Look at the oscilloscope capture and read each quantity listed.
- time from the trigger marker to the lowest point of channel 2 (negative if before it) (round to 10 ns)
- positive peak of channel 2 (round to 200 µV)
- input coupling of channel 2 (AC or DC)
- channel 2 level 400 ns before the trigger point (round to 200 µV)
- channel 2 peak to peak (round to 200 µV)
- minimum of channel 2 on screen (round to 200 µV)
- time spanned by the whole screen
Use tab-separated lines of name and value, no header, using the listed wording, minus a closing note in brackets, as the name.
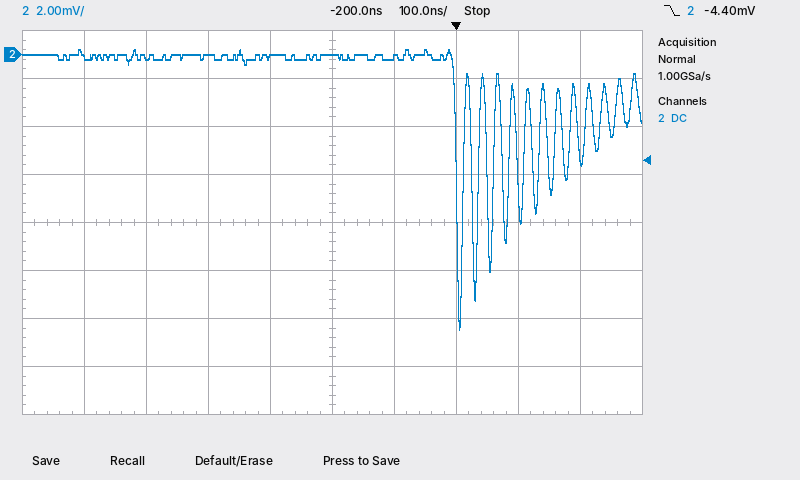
time from the trigger marker to the lowest point of channel 2 (negative if before it)	+10 ns
positive peak of channel 2	200 µV
input coupling of channel 2	DC
channel 2 level 400 ns before the trigger point	0.0 mV
channel 2 peak to peak	11.6 mV
minimum of channel 2 on screen	-11.4 mV
time spanned by the whole screen	1 µs
